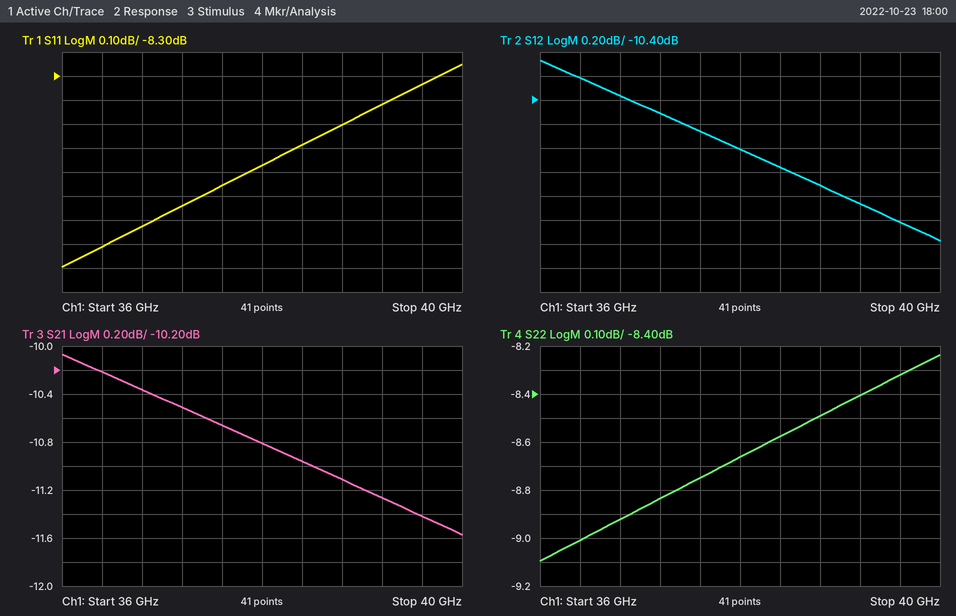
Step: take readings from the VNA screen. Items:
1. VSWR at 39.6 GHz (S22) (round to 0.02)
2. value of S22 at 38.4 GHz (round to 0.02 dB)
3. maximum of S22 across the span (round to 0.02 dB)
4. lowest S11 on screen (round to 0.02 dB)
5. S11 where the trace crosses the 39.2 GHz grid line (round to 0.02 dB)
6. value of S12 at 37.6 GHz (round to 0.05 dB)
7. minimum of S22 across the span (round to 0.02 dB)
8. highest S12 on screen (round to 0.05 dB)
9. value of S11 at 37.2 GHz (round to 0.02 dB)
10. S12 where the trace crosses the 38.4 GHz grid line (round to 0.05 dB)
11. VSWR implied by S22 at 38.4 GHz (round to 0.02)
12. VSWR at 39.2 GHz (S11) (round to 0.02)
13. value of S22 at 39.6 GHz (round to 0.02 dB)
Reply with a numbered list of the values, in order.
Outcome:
1. 2.24
2. -8.58 dB
3. -8.24 dB
4. -9.10 dB
5. -8.42 dB
6. -10.65 dB
7. -9.10 dB
8. -10.05 dB
9. -8.84 dB
10. -10.95 dB
11. 2.18
12. 2.22
13. -8.32 dB
